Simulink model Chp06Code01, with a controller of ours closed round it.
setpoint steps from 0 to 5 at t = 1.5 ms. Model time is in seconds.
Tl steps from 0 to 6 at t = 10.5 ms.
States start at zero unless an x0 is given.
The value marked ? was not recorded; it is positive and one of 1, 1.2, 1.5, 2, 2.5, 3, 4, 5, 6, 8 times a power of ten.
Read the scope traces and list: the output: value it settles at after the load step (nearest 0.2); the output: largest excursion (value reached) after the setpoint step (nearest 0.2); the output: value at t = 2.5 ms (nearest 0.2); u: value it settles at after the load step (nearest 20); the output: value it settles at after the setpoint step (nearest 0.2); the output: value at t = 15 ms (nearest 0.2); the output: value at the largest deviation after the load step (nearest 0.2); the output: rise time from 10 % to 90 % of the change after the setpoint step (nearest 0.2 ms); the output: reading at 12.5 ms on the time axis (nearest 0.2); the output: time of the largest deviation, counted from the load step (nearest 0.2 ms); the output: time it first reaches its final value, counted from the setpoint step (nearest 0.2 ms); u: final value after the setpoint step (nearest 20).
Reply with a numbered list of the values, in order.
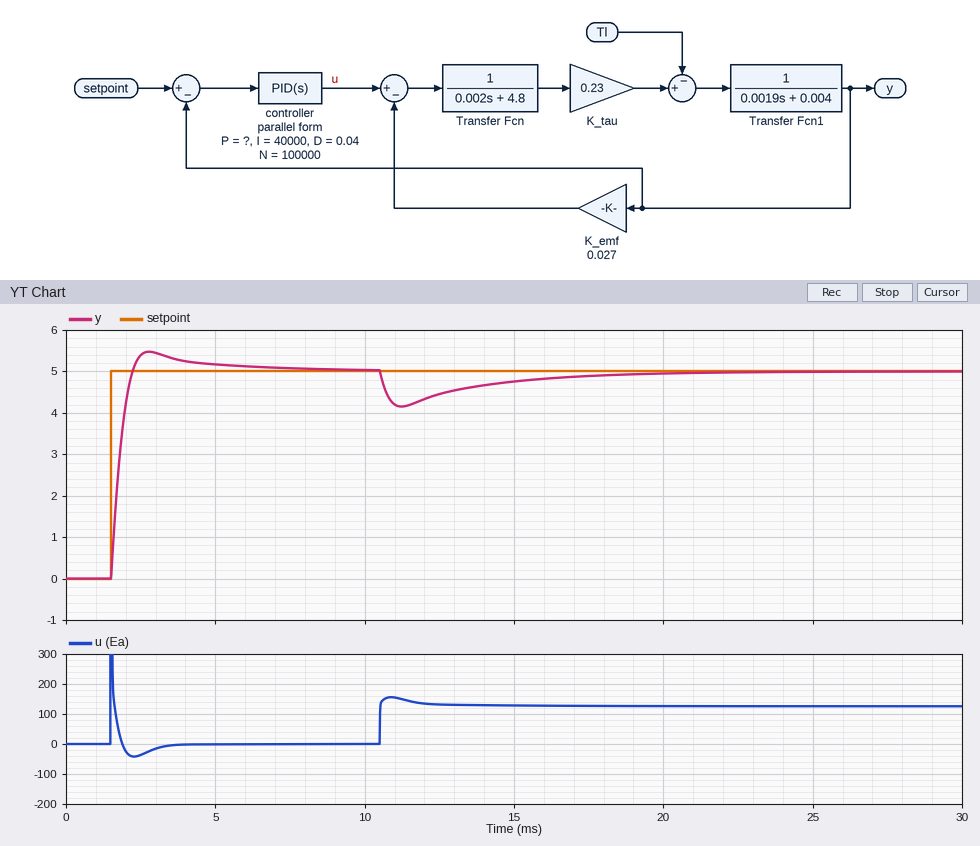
1. 5.0
2. 5.4
3. 5.4
4. 120
5. 5.0
6. 4.8
7. 4.2
8. 0.6 ms
9. 4.4
10. 0.8 ms
11. 0.8 ms
12. 0
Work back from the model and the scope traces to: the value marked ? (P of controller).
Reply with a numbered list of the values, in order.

1. 150
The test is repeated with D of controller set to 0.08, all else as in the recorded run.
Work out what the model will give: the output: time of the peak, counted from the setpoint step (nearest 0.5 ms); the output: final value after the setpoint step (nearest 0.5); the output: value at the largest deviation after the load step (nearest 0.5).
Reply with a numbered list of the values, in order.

1. 2.5 ms
2. 5.0
3. 4.5
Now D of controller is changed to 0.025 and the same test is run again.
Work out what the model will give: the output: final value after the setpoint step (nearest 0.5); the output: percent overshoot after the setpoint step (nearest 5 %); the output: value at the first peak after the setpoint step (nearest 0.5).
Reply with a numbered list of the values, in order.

1. 5.0
2. 15 %
3. 6.0
